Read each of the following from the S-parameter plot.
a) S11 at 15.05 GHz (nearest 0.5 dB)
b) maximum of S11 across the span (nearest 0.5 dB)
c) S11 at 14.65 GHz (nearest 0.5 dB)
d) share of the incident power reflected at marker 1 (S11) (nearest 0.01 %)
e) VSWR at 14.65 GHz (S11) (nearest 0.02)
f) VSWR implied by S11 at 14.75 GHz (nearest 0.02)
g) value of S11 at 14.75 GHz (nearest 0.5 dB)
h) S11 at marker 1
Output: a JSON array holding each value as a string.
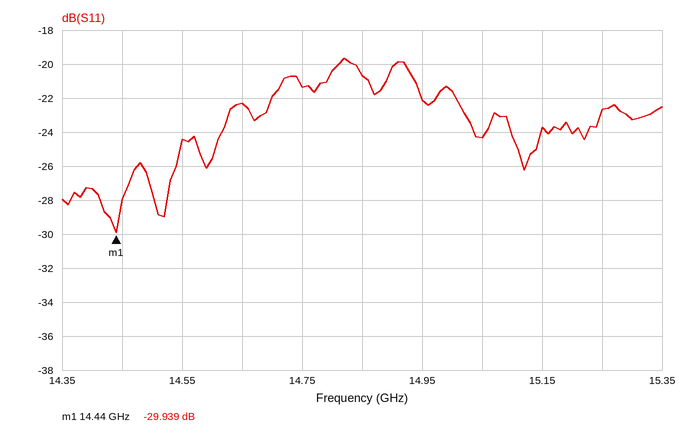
["-24.5 dB", "-19.5 dB", "-22.5 dB", "0.10 %", "1.16", "1.18", "-21.5 dB", "-29.939 dB"]
